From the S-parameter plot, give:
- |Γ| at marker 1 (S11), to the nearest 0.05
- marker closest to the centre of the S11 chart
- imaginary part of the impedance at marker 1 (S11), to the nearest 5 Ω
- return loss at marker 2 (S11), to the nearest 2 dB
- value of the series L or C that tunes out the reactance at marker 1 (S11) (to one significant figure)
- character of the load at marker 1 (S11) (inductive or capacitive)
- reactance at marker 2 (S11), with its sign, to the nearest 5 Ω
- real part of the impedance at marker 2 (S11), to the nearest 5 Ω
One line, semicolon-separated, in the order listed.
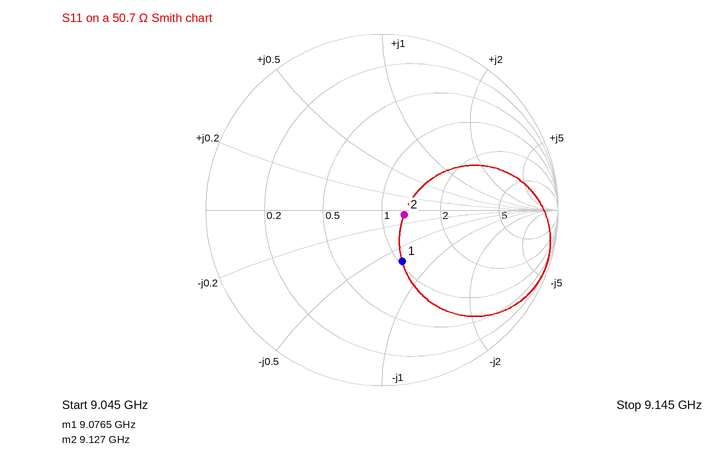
0.30; marker 2; -35 Ω; 18 dB; 600 pH; capacitive; -5 Ω; 65 Ω
